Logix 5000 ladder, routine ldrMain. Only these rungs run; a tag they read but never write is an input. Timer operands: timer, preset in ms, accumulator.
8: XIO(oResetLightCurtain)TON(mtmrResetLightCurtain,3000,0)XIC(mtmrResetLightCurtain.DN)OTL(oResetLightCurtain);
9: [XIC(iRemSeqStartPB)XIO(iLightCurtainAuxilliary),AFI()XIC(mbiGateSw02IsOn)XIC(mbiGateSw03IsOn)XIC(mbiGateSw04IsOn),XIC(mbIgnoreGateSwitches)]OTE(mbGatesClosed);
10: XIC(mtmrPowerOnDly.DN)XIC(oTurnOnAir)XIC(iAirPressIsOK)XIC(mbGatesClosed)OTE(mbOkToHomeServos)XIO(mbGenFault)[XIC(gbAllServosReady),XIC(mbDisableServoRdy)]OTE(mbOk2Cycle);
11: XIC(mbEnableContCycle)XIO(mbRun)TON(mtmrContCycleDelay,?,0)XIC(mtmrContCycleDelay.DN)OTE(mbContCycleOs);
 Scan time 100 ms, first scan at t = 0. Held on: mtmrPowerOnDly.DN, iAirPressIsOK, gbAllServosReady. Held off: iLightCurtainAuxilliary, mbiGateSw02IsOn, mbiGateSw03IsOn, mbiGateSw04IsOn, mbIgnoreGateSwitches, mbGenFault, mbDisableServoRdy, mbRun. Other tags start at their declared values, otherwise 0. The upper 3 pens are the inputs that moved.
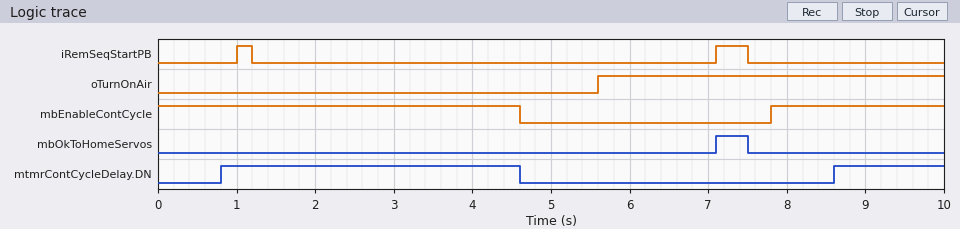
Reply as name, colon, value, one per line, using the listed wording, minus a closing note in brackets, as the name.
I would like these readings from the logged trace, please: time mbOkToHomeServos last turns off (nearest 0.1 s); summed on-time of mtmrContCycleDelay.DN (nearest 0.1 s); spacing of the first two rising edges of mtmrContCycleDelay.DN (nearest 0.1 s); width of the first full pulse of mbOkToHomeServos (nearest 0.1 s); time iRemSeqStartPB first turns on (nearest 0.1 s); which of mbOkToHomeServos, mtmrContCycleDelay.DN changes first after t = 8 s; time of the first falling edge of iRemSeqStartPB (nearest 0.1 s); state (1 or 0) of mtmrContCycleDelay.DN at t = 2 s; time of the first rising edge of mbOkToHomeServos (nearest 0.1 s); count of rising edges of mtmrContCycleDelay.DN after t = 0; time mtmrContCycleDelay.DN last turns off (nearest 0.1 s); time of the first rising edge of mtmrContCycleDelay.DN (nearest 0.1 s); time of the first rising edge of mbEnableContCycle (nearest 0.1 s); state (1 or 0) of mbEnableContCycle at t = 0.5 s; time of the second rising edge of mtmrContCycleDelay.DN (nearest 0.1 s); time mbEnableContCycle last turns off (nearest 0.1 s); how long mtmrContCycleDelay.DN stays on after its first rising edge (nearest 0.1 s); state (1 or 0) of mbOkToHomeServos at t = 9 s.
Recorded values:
time mbOkToHomeServos last turns off: 7.5 s
summed on-time of mtmrContCycleDelay.DN: 5.2 s
spacing of the first two rising edges of mtmrContCycleDelay.DN: 7.8 s
width of the first full pulse of mbOkToHomeServos: 0.4 s
time iRemSeqStartPB first turns on: 1.0 s
which of mbOkToHomeServos, mtmrContCycleDelay.DN changes first after t = 8 s: mtmrContCycleDelay.DN
time of the first falling edge of iRemSeqStartPB: 1.2 s
state (1 or 0) of mtmrContCycleDelay.DN at t = 2 s: 1
time of the first rising edge of mbOkToHomeServos: 7.1 s
count of rising edges of mtmrContCycleDelay.DN after t = 0: 2
time mtmrContCycleDelay.DN last turns off: 4.6 s
time of the first rising edge of mtmrContCycleDelay.DN: 0.8 s
time of the first rising edge of mbEnableContCycle: 7.8 s
state (1 or 0) of mbEnableContCycle at t = 0.5 s: 1
time of the second rising edge of mtmrContCycleDelay.DN: 8.6 s
time mbEnableContCycle last turns off: 4.6 s
how long mtmrContCycleDelay.DN stays on after its first rising edge: 3.8 s
state (1 or 0) of mbOkToHomeServos at t = 9 s: 0
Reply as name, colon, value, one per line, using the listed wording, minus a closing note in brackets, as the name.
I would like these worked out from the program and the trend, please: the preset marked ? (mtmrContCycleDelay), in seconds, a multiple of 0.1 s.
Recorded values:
the preset marked ? (mtmrContCycleDelay), in seconds, a multiple of 0.1 s: 0.8 s
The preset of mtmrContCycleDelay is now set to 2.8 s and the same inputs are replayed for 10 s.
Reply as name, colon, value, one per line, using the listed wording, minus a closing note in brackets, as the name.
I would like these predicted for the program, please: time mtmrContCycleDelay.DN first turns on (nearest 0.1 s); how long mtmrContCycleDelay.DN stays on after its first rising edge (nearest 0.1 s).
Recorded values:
time mtmrContCycleDelay.DN first turns on: 2.8 s
how long mtmrContCycleDelay.DN stays on after its first rising edge: 1.8 s
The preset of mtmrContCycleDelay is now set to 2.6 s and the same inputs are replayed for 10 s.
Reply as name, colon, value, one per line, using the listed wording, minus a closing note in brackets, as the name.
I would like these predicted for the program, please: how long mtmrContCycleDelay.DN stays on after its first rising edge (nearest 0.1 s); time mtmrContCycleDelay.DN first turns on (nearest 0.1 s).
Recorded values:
how long mtmrContCycleDelay.DN stays on after its first rising edge: 2.0 s
time mtmrContCycleDelay.DN first turns on: 2.6 s
